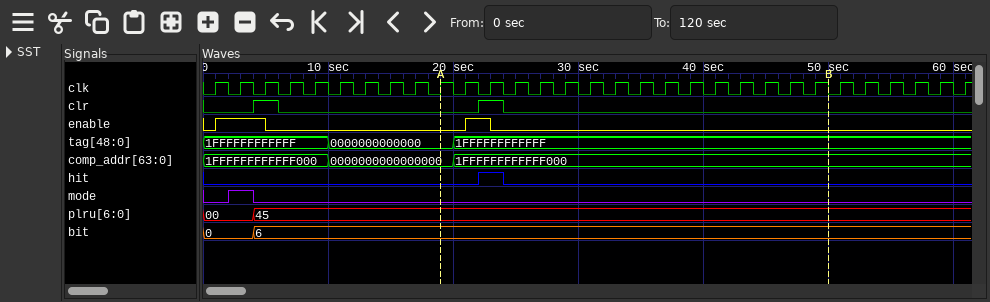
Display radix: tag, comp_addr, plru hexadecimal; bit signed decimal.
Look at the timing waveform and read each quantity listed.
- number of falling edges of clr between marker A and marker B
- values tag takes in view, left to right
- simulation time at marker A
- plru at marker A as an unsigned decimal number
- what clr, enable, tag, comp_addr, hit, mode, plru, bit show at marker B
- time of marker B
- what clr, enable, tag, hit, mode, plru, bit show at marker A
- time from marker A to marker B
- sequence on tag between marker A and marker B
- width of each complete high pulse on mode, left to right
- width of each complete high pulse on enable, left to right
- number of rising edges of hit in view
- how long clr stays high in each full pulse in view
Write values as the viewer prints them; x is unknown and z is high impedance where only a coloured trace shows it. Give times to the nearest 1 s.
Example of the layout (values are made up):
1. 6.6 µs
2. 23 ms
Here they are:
1. 1
2. 1FFFFFFFFFFFF, 0000000000000, 1FFFFFFFFFFFF
3. 19 s
4. 69
5. clr=0, enable=0, tag=1FFFFFFFFFFFF, comp_addr=1FFFFFFFFFFFF000, hit=0, mode=0, plru=45, bit=6
6. 50 s
7. clr=0, enable=0, tag=0000000000000, hit=0, mode=0, plru=45, bit=6
8. 31 s
9. 0000000000000, 1FFFFFFFFFFFF
10. 2 s
11. 4 s, 2 s
12. 1
13. 2 s, 2 s
